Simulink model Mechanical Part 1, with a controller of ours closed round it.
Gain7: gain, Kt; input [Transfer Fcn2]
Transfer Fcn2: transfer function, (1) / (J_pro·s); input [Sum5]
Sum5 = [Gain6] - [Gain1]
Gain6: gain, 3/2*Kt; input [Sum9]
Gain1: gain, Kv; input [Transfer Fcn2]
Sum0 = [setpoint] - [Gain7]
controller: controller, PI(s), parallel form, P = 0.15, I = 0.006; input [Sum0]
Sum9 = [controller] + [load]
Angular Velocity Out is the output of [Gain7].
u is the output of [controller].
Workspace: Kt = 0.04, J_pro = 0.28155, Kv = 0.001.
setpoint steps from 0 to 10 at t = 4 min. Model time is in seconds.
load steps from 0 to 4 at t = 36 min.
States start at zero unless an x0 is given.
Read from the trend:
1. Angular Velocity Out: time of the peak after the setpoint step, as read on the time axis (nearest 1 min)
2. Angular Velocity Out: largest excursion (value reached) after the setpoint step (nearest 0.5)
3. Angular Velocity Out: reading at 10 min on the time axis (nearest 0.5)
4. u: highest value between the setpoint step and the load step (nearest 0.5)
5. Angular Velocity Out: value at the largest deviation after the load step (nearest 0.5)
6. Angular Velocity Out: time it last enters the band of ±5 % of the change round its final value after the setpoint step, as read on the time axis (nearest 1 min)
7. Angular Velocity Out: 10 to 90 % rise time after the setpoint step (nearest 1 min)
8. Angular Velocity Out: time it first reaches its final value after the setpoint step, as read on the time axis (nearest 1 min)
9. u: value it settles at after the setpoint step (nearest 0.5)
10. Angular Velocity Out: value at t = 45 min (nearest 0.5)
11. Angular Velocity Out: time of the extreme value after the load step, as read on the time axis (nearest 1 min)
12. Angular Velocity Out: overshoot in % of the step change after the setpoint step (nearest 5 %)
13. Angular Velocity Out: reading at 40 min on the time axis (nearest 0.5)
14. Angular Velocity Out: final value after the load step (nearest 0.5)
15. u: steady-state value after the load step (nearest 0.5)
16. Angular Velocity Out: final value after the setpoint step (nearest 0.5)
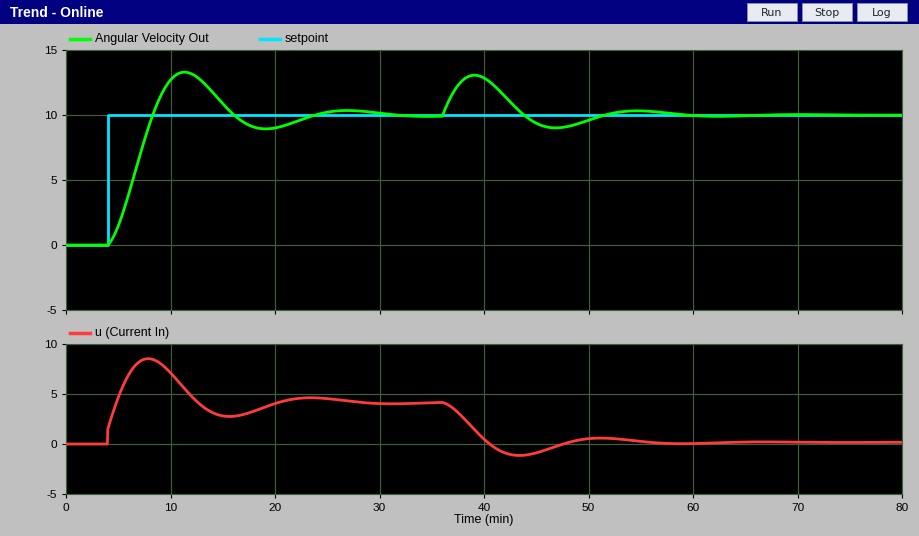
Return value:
11 min
13.5
12.5
8.5
13.0
22 min
3 min
8 min
4.0
9.5
39 min
35 %
13.0
10.0
0.0
10.0
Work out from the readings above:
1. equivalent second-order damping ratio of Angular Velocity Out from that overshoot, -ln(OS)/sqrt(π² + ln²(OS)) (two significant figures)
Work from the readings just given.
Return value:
0.32
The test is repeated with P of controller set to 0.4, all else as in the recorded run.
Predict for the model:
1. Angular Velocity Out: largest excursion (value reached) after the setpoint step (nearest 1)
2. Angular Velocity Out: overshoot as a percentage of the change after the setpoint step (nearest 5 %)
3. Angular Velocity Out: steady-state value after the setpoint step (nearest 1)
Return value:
12
20 %
10
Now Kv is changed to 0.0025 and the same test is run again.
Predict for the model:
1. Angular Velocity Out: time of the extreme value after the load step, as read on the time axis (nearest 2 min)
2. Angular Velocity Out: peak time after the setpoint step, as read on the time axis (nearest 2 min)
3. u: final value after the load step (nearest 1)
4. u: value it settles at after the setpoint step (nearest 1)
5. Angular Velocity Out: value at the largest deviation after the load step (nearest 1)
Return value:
38 min
14 min
6
10
12
